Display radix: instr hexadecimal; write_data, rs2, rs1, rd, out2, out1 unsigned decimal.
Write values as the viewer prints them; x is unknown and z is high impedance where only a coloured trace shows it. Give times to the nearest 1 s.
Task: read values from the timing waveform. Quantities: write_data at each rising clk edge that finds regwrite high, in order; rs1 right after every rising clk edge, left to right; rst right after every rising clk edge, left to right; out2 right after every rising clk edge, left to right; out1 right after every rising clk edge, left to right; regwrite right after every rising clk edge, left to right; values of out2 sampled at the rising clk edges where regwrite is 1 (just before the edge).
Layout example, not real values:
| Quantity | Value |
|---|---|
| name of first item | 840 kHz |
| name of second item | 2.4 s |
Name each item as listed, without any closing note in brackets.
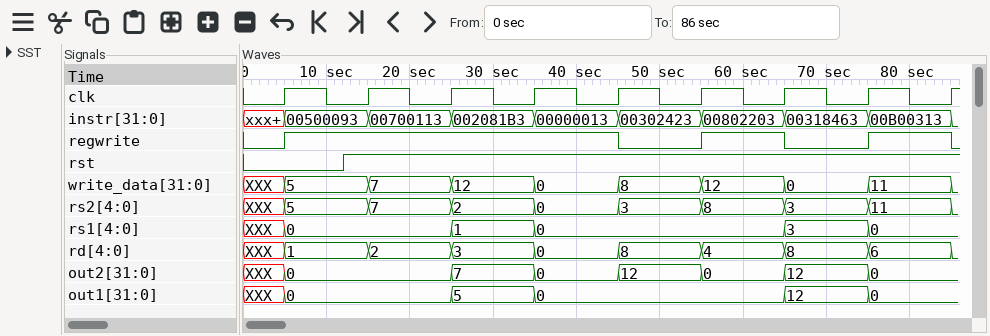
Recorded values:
| Quantity | Value |
|---|---|
| write_data at each rising clk edge that finds regwrite high, in order | 5, 7, 12, 0, 12, 11 |
| rs1 right after every rising clk edge, left to right | 0, 0, 1, 0, 0, 0, 3, 0, 0 |
| rst right after every rising clk edge, left to right | 0 1 1 1 1 1 1 1 1 |
| out2 right after every rising clk edge, left to right | 0, 0, 7, 0, 12, 0, 12, 0, 0 |
| out1 right after every rising clk edge, left to right | 0, 0, 5, 0, 0, 0, 12, 0, 0 |
| regwrite right after every rising clk edge, left to right | 1 1 1 1 0 1 0 1 0 |
| values of out2 sampled at the rising clk edges where regwrite is 1 | 0, 0, 7, 0, 0, 0 |
